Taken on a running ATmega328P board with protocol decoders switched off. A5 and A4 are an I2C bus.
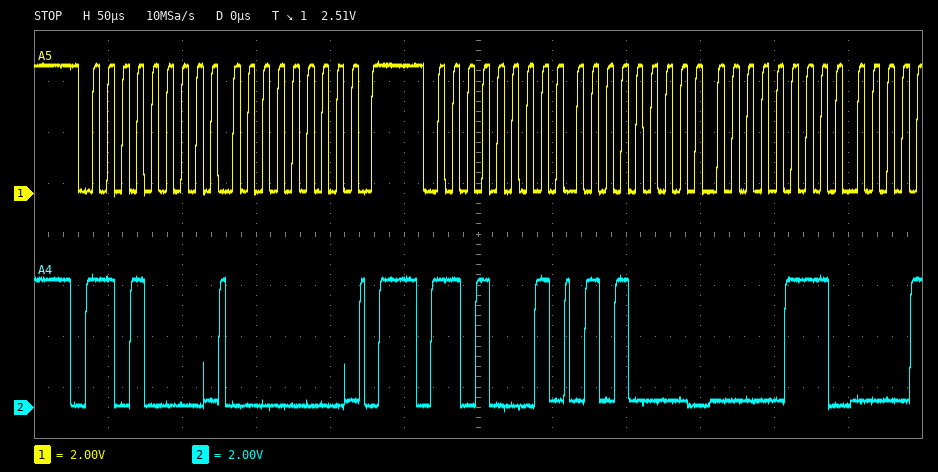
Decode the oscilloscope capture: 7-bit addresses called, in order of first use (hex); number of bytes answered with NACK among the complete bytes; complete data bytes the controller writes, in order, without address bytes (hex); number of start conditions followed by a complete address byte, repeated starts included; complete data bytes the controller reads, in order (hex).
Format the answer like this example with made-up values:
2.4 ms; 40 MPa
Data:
0x68; 0; 00; 2; 50 07
